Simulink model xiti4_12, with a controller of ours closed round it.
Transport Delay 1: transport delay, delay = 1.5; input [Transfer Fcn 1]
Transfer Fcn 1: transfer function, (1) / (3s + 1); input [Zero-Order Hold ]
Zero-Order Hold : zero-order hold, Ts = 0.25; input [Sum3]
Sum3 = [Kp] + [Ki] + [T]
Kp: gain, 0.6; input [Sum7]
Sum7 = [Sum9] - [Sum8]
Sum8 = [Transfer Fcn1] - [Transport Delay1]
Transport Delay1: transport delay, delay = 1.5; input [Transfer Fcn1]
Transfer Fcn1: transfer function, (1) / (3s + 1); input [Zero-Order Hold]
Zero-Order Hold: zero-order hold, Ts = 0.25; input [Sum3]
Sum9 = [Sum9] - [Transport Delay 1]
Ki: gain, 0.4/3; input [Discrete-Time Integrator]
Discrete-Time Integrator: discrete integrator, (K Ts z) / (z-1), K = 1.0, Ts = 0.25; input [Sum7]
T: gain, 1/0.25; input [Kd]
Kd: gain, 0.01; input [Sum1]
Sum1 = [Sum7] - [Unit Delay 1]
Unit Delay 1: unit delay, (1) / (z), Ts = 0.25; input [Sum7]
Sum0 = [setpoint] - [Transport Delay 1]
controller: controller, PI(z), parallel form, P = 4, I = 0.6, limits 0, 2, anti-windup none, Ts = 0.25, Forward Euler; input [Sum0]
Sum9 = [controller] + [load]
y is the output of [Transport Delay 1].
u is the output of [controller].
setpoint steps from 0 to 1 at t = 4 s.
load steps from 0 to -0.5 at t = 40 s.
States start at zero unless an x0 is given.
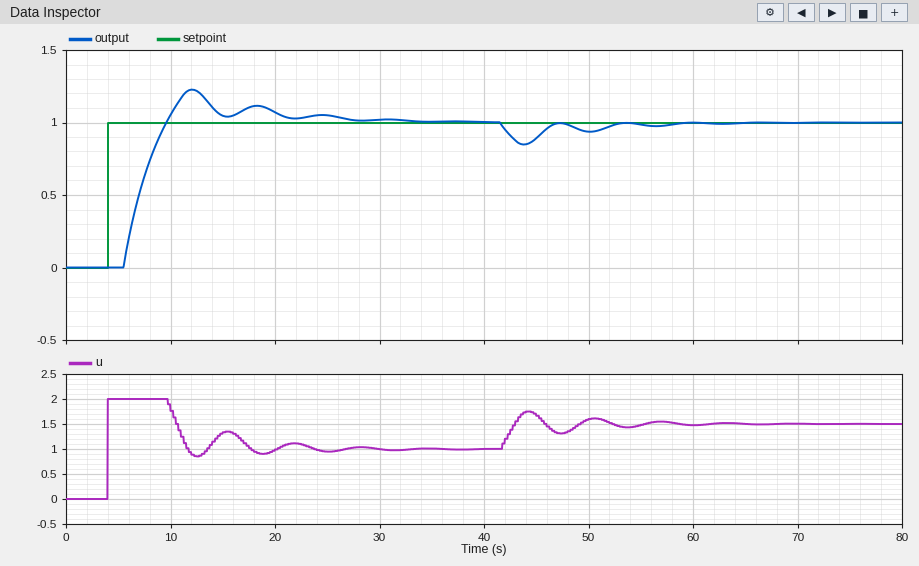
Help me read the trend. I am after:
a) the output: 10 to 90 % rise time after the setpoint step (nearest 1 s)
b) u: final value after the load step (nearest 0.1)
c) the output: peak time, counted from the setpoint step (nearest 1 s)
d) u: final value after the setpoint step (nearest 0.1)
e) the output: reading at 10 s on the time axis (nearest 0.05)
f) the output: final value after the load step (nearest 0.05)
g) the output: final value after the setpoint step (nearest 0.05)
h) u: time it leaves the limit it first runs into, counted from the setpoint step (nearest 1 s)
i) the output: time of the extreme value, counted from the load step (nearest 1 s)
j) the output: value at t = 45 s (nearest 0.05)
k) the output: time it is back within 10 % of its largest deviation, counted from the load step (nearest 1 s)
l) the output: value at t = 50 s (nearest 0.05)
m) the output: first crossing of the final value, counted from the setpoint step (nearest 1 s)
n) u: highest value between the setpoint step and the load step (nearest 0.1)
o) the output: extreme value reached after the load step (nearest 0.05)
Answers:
3 s
1.5
8 s
1.0
1.05
1.00
1.00
6 s
4 s
0.90
18 s
0.95
6 s
2.0
0.85
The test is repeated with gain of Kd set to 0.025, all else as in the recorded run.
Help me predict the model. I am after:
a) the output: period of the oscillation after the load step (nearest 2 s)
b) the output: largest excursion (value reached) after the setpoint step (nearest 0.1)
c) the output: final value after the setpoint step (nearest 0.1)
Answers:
6 s
1.2
1.0
